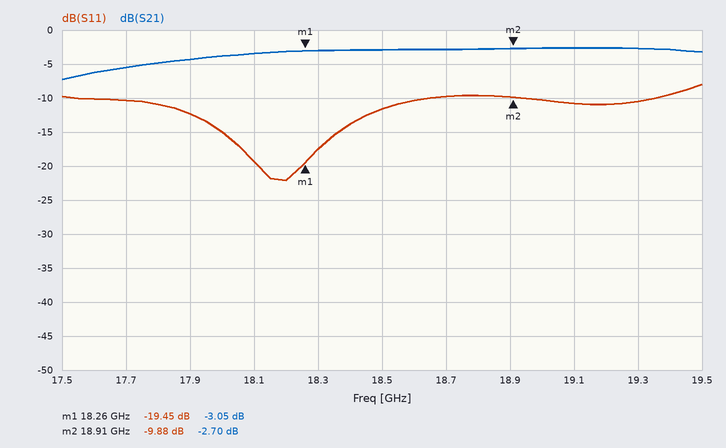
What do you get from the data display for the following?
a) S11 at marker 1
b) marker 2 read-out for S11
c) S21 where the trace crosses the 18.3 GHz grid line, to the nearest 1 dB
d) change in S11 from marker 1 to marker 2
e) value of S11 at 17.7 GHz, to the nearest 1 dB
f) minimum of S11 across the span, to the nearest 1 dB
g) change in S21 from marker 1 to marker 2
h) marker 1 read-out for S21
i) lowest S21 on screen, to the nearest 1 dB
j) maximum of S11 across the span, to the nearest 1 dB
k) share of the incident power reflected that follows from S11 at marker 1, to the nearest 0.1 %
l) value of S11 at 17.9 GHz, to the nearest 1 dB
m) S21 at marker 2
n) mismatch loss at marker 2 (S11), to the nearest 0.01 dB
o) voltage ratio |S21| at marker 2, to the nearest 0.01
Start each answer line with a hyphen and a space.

- -19.45 dB
- -9.88 dB
- -3 dB
- 9.57 dB
- -10 dB
- -22 dB
- 0.35 dB
- -3.05 dB
- -7 dB
- -8 dB
- 1.1 %
- -12 dB
- -2.70 dB
- 0.47 dB
- 0.73
